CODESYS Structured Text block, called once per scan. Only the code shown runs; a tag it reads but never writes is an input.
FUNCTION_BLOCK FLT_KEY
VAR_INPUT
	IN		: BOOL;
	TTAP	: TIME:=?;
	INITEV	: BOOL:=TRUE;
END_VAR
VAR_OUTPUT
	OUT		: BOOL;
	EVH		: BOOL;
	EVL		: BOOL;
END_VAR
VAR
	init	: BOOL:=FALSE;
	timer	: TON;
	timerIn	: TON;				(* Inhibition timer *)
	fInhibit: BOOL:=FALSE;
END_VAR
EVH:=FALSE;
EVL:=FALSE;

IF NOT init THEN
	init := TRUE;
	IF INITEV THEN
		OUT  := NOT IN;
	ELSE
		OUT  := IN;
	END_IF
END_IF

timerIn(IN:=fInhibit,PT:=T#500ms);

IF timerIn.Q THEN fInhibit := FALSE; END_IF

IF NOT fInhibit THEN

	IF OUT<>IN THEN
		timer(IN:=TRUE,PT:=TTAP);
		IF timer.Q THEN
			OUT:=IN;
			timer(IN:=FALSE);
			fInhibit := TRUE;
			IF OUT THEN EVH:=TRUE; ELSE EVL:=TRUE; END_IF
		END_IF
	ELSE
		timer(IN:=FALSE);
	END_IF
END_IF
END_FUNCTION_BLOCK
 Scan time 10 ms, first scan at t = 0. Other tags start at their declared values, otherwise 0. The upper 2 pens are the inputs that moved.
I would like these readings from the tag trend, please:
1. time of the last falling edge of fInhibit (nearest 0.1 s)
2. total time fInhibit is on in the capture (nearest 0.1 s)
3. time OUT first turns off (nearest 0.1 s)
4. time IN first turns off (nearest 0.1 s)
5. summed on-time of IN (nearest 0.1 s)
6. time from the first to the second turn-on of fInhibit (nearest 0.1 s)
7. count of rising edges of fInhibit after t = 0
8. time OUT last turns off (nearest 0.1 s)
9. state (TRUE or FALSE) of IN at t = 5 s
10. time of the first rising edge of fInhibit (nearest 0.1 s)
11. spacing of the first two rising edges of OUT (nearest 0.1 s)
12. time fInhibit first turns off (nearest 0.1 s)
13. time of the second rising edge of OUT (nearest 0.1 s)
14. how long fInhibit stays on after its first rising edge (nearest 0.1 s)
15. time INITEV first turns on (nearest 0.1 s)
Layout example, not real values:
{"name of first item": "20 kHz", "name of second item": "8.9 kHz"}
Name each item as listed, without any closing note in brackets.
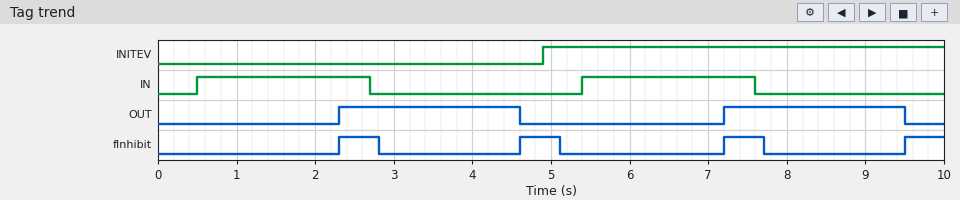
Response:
{"time of the last falling edge of fInhibit": "7.7 s", "total time fInhibit is on in the capture": "2.0 s", "time OUT first turns off": "4.6 s", "time IN first turns off": "2.7 s", "summed on-time of IN": "4.4 s", "time from the first to the second turn-on of fInhibit": "2.3 s", "count of rising edges of fInhibit after t = 0": "4", "time OUT last turns off": "9.5 s", "state (TRUE or FALSE) of IN at t = 5 s": "FALSE", "time of the first rising edge of fInhibit": "2.3 s", "spacing of the first two rising edges of OUT": "4.9 s", "time fInhibit first turns off": "2.8 s", "time of the second rising edge of OUT": "7.2 s", "how long fInhibit stays on after its first rising edge": "0.5 s", "time INITEV first turns on": "4.9 s"}
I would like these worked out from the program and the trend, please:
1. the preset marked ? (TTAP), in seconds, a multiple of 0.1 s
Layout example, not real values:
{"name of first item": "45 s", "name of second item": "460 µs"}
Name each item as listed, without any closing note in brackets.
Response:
{"the preset marked ? (TTAP), in seconds, a multiple of 0.1 s": "1.8 s"}
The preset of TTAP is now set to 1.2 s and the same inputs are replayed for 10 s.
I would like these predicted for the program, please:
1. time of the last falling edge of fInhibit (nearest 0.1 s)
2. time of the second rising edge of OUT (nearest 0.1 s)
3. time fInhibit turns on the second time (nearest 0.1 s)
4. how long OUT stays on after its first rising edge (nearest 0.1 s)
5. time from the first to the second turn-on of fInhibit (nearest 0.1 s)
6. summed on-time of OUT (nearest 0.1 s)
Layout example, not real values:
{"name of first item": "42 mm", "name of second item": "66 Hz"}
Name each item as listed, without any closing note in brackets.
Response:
{"time of the last falling edge of fInhibit": "9.3 s", "time of the second rising edge of OUT": "6.6 s", "time fInhibit turns on the second time": "3.9 s", "how long OUT stays on after its first rising edge": "2.2 s", "time from the first to the second turn-on of fInhibit": "2.2 s", "summed on-time of OUT": "4.4 s"}
